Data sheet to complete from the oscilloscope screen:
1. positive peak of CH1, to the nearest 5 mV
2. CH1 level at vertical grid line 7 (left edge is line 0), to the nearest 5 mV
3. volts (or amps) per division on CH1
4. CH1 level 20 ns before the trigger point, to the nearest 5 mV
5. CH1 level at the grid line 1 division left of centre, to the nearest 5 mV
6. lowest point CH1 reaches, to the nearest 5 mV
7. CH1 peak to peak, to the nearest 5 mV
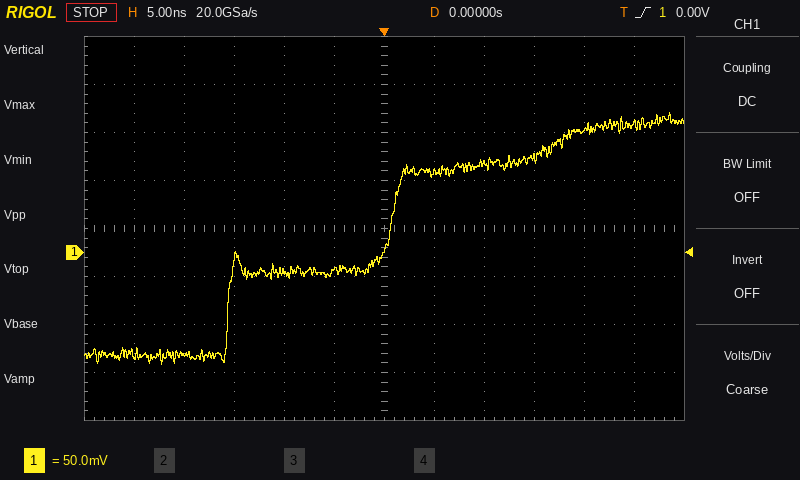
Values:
145 mV
85 mV
50 mV
-105 mV
-20 mV
-115 mV
260 mV
